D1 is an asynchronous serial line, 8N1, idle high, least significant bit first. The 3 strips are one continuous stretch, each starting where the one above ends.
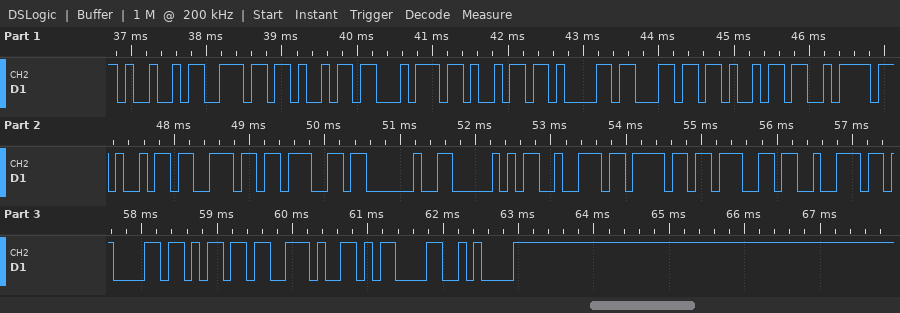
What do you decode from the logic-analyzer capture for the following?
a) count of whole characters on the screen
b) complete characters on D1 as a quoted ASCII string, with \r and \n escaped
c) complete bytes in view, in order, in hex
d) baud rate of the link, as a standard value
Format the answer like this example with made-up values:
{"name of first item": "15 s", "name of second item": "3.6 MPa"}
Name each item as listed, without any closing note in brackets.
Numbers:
{"count of whole characters on the screen": "23", "complete characters on D1 as a quoted ASCII string, with \\r and \\n escaped": "\"Initializing Program.\\r\\n\"", "complete bytes in view, in order, in hex": "49 6E 69 74 69 61 6C 69 7A 69 6E 67 20 50 72 6F 67 72 61 6D 2E 0D 0A", "baud rate of the link, as a standard value": "9600 baud"}
